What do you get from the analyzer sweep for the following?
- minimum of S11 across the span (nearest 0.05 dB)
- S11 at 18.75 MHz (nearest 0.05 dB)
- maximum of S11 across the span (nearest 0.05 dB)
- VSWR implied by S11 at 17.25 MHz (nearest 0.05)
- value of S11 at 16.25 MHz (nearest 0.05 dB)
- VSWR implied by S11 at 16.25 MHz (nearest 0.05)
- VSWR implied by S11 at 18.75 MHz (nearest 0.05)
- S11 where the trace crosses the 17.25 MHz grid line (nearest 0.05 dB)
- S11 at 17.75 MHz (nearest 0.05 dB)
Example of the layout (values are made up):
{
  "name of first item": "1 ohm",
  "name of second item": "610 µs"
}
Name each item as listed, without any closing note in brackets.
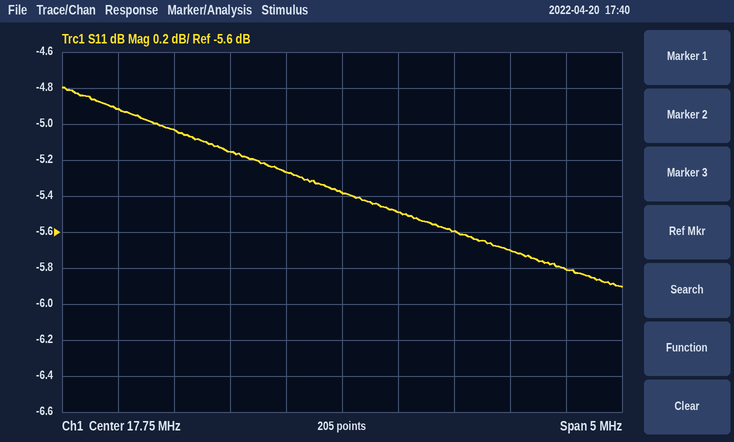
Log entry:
{
  "minimum of S11 across the span": "-5.90 dB",
  "S11 at 18.75 MHz": "-5.60 dB",
  "maximum of S11 across the span": "-4.80 dB",
  "VSWR implied by S11 at 17.25 MHz": "3.40",
  "value of S11 at 16.25 MHz": "-5.05 dB",
  "VSWR implied by S11 at 16.25 MHz": "3.55",
  "VSWR implied by S11 at 18.75 MHz": "3.20",
  "S11 where the trace crosses the 17.25 MHz grid line": "-5.25 dB",
  "S11 at 17.75 MHz": "-5.40 dB"
}
